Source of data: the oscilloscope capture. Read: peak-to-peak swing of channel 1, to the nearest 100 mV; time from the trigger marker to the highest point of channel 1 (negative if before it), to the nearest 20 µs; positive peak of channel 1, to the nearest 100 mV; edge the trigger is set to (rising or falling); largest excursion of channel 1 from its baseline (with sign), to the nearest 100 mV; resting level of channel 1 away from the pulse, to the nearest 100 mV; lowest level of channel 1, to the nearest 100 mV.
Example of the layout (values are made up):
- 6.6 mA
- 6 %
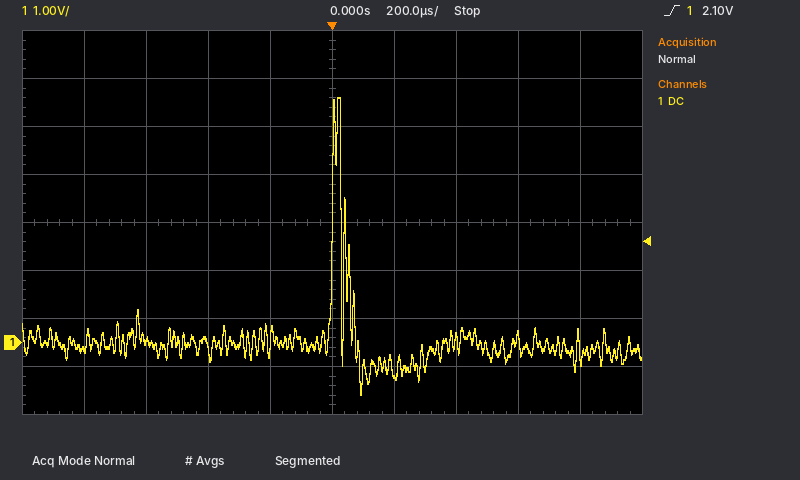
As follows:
- 6.2 V
- +20 µs
- 5.1 V
- rising
- +5.2 V
- -100 mV
- -1.1 V
